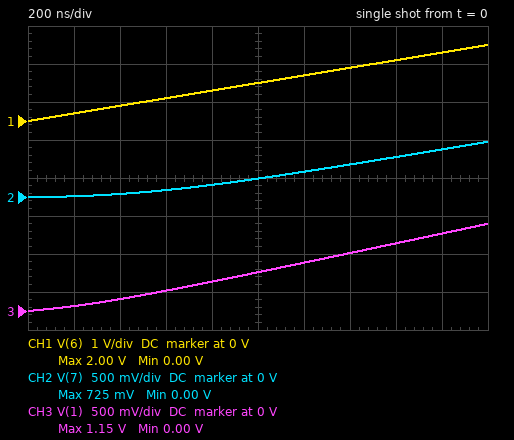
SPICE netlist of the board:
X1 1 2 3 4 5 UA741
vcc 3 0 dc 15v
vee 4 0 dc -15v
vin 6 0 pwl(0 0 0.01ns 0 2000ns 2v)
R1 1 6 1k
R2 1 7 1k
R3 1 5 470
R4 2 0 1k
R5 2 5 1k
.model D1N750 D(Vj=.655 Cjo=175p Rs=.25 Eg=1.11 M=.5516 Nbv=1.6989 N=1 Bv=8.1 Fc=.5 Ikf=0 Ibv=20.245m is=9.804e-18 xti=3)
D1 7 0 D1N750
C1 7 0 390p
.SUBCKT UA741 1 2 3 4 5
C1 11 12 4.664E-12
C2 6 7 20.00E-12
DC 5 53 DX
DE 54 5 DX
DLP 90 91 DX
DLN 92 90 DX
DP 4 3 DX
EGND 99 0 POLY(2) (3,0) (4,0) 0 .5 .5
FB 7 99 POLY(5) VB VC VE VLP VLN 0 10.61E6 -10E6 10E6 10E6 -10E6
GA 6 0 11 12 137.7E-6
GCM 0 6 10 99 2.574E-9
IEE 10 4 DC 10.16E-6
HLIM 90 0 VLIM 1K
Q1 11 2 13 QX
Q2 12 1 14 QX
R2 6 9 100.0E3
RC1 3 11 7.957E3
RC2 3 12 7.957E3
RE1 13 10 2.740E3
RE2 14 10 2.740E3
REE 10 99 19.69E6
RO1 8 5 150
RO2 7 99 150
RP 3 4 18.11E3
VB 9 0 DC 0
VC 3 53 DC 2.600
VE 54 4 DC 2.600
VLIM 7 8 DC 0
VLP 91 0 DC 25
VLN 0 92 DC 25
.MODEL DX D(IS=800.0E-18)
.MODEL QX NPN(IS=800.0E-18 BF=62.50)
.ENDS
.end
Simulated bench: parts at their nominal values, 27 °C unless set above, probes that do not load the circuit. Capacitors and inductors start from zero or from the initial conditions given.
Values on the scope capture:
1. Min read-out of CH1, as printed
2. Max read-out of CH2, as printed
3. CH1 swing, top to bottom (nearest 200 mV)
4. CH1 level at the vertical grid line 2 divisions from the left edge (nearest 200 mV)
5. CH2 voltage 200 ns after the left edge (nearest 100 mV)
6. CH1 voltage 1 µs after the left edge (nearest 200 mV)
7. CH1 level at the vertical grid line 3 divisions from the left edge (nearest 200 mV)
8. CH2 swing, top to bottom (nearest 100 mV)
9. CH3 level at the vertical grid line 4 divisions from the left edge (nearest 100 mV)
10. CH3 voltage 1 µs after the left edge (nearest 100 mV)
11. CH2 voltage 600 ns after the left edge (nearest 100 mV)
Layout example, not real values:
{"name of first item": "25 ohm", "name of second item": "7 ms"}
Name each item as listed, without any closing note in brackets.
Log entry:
{"Min read-out of CH1, as printed": "0.00 V", "Max read-out of CH2, as printed": "725 mV", "CH1 swing, top to bottom": "2.0 V", "CH1 level at the vertical grid line 2 divisions from the left edge": "400 mV", "CH2 voltage 200 ns after the left edge": "0 V", "CH1 voltage 1 µs after the left edge": "1.0 V", "CH1 level at the vertical grid line 3 divisions from the left edge": "600 mV", "CH2 swing, top to bottom": "700 mV", "CH3 level at the vertical grid line 4 divisions from the left edge": "400 mV", "CH3 voltage 1 µs after the left edge": "500 mV", "CH2 voltage 600 ns after the left edge": "100 mV"}
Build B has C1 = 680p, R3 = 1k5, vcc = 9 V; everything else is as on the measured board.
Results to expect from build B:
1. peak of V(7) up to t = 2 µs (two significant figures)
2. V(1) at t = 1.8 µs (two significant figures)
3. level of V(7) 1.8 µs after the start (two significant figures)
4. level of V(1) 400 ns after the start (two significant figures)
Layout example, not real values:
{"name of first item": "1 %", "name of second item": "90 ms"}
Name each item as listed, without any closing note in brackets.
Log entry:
{"peak of V(7) up to t = 2 µs": "680 mV", "V(1) at t = 1.8 µs": "1.1 V", "level of V(7) 1.8 µs after the start": "580 mV", "level of V(1) 400 ns after the start": "190 mV"}
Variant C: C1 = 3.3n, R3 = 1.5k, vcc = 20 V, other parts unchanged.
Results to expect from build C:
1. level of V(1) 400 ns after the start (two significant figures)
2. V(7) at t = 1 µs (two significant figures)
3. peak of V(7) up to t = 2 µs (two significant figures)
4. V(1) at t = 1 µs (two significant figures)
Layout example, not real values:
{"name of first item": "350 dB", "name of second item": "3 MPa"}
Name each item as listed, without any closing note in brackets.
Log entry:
{"level of V(1) 400 ns after the start": "180 mV", "V(7) at t = 1 µs": "62 mV", "peak of V(7) up to t = 2 µs": "240 mV", "V(1) at t = 1 µs": "500 mV"}
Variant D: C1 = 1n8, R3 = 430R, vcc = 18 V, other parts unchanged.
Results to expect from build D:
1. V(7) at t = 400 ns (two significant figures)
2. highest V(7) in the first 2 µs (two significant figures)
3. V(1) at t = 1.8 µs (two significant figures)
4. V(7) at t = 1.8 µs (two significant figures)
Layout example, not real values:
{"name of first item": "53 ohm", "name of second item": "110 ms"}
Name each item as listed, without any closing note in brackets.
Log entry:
{"V(7) at t = 400 ns": "12 mV", "highest V(7) in the first 2 µs": "350 mV", "V(1) at t = 1.8 µs": "920 mV", "V(7) at t = 1.8 µs": "290 mV"}
